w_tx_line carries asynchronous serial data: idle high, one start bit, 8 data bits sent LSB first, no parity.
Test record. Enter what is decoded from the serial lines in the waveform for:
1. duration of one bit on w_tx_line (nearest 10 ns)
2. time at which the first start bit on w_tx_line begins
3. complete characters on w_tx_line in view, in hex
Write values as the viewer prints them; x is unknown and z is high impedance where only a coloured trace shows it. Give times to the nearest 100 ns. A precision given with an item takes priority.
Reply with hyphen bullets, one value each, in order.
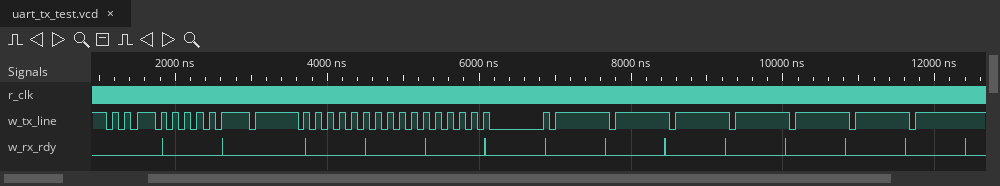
- 80 ns
- 1100 ns
- 75, 55, 7F, 55, 55, 55, 00, FF, FF, FF, FF, FF, FF, FF
